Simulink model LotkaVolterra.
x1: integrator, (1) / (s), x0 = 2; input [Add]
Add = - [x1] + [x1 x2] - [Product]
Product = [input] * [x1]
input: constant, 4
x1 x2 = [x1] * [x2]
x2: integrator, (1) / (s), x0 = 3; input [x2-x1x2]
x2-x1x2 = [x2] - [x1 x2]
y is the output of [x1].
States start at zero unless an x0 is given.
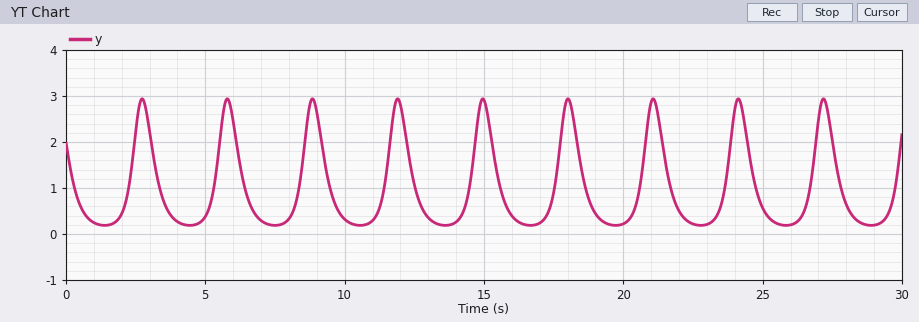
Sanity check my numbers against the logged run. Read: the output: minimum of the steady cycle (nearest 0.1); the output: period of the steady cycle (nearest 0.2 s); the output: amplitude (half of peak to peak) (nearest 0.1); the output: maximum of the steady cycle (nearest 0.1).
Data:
0.2
3.0 s
1.4
2.9
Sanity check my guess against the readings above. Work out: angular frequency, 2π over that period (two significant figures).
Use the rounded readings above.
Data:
2.1 rad/s
